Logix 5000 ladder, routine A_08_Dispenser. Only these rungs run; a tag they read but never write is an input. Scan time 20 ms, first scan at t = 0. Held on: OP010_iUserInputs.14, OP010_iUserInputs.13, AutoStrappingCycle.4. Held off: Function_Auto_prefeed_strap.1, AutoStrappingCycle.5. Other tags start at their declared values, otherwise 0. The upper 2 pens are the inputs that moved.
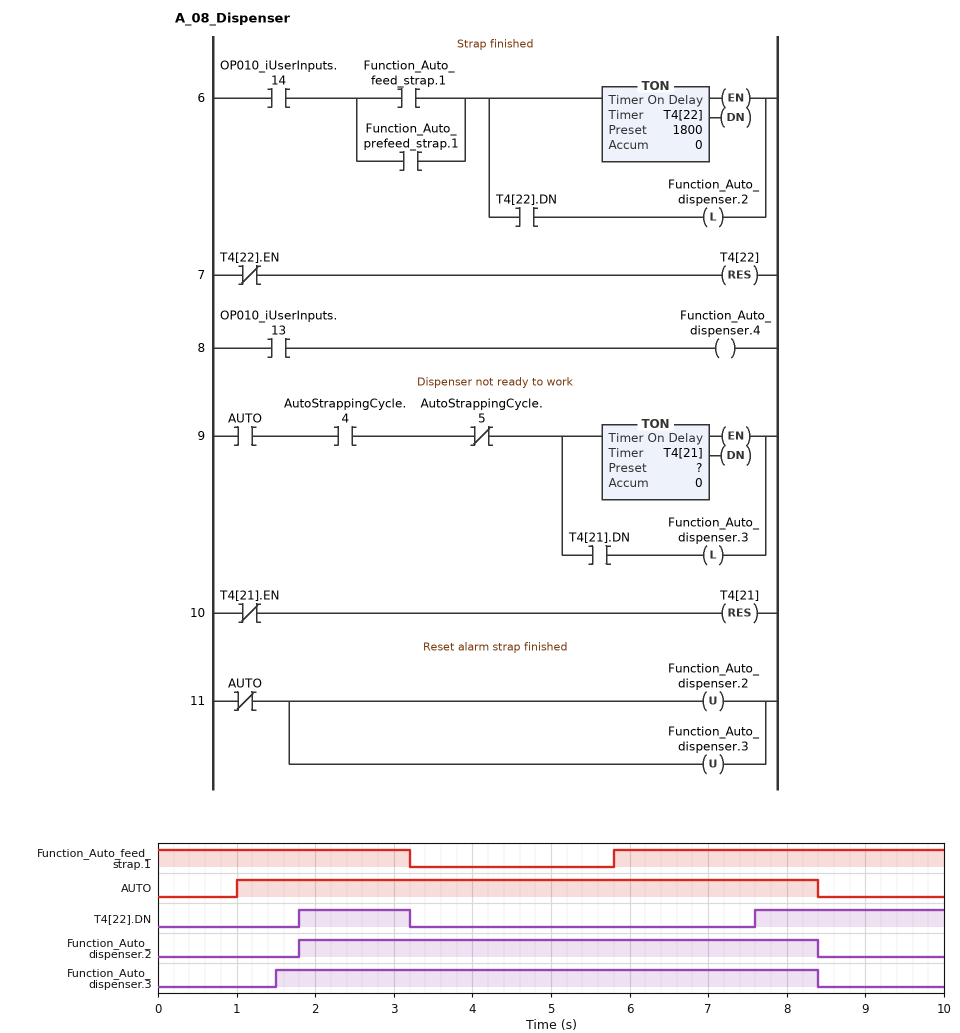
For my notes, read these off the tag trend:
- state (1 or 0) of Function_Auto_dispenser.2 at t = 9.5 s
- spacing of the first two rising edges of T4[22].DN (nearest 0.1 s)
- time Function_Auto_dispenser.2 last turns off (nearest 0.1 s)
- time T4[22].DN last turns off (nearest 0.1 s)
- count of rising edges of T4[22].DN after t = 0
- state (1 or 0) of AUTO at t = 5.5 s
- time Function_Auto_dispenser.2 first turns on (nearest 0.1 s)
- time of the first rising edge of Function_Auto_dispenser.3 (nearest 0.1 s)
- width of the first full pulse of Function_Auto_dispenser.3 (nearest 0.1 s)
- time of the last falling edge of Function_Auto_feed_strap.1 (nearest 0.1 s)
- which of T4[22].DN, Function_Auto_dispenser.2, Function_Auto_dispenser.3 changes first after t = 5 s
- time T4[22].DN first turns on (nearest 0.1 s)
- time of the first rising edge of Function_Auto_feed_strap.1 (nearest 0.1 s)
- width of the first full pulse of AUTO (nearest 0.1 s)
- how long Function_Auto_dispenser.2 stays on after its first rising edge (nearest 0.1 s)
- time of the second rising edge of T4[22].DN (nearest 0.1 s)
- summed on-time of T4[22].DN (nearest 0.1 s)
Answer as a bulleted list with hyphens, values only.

- 0
- 5.8 s
- 8.4 s
- 3.2 s
- 2
- 1
- 1.8 s
- 1.5 s
- 6.9 s
- 3.2 s
- T4[22].DN
- 1.8 s
- 5.8 s
- 7.4 s
- 6.6 s
- 7.6 s
- 3.8 s
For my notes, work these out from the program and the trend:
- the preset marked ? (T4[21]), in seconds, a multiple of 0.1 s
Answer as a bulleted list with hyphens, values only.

- 0.5 s
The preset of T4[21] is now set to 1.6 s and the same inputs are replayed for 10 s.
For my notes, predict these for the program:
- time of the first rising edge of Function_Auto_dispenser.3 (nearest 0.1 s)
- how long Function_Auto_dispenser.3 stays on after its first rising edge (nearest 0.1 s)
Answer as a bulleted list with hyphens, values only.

- 2.6 s
- 5.8 s
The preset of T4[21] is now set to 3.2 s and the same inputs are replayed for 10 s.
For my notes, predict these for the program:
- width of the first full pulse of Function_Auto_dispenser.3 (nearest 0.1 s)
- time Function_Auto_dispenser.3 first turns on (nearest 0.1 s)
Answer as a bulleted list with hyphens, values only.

- 4.2 s
- 4.2 s
